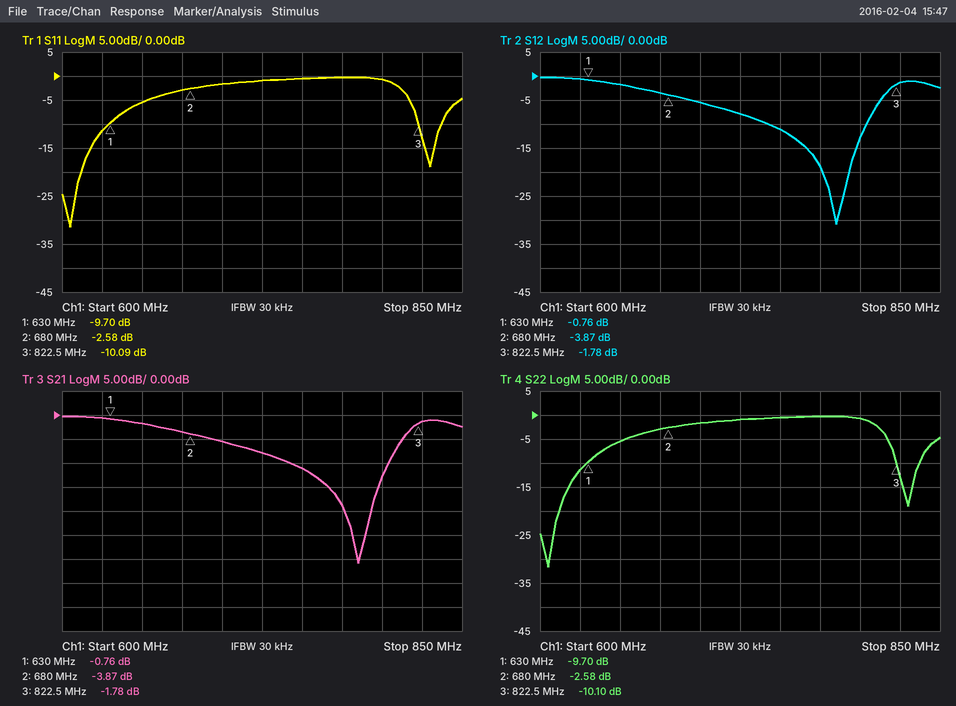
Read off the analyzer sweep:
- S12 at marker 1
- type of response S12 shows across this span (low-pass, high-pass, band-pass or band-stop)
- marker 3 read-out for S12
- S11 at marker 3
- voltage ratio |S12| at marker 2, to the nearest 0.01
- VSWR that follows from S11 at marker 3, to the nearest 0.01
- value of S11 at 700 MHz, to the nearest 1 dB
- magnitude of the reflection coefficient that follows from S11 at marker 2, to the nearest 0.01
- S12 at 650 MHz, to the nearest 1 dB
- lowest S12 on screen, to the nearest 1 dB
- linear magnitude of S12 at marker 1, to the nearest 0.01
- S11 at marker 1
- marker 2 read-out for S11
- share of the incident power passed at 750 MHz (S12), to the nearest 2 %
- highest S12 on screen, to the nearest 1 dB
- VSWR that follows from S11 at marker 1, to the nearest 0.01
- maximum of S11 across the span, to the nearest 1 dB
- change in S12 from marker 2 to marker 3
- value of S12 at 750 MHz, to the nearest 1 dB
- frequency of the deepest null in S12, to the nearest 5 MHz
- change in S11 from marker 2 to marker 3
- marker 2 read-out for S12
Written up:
-0.76 dB
band-stop
-1.78 dB
-10.09 dB
0.64
1.91
-2 dB
0.74
-2 dB
-31 dB
0.92
-9.70 dB
-2.58 dB
8 %
0 dB
1.97
0 dB
2.09 dB
-11 dB
785 MHz
-7.51 dB
-3.87 dB
